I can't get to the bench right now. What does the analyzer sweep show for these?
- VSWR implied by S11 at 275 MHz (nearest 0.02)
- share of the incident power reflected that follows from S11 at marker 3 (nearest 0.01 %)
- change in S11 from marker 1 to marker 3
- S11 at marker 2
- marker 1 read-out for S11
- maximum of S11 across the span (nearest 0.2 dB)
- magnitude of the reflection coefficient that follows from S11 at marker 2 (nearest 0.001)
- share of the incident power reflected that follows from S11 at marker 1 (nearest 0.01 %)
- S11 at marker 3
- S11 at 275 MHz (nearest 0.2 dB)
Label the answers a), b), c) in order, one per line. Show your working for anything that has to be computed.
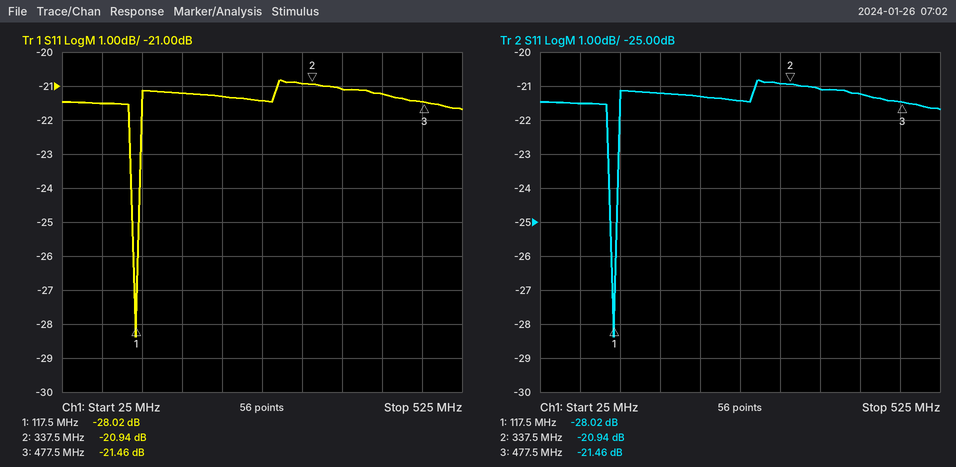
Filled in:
a) |Γ| = 10^(-21.4/20) = 0.0851; VSWR = (1 + 0.0851)/(1 − 0.0851) ≈ 1.19, so 1.18 to the nearest 0.02
b) 10^(-21.46/10) ≈ 0.71 %
c) -21.46 − (-28.02) = 6.56 dB
d) -20.94 dB
e) -28.02 dB
f) -20.8 dB
g) 10^(-20.94/20) ≈ 0.090
h) 10^(-28.02/10) ≈ 0.16 %
i) -21.46 dB
j) -21.4 dB
